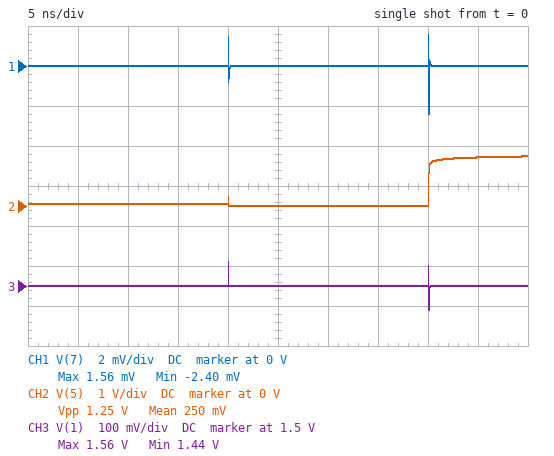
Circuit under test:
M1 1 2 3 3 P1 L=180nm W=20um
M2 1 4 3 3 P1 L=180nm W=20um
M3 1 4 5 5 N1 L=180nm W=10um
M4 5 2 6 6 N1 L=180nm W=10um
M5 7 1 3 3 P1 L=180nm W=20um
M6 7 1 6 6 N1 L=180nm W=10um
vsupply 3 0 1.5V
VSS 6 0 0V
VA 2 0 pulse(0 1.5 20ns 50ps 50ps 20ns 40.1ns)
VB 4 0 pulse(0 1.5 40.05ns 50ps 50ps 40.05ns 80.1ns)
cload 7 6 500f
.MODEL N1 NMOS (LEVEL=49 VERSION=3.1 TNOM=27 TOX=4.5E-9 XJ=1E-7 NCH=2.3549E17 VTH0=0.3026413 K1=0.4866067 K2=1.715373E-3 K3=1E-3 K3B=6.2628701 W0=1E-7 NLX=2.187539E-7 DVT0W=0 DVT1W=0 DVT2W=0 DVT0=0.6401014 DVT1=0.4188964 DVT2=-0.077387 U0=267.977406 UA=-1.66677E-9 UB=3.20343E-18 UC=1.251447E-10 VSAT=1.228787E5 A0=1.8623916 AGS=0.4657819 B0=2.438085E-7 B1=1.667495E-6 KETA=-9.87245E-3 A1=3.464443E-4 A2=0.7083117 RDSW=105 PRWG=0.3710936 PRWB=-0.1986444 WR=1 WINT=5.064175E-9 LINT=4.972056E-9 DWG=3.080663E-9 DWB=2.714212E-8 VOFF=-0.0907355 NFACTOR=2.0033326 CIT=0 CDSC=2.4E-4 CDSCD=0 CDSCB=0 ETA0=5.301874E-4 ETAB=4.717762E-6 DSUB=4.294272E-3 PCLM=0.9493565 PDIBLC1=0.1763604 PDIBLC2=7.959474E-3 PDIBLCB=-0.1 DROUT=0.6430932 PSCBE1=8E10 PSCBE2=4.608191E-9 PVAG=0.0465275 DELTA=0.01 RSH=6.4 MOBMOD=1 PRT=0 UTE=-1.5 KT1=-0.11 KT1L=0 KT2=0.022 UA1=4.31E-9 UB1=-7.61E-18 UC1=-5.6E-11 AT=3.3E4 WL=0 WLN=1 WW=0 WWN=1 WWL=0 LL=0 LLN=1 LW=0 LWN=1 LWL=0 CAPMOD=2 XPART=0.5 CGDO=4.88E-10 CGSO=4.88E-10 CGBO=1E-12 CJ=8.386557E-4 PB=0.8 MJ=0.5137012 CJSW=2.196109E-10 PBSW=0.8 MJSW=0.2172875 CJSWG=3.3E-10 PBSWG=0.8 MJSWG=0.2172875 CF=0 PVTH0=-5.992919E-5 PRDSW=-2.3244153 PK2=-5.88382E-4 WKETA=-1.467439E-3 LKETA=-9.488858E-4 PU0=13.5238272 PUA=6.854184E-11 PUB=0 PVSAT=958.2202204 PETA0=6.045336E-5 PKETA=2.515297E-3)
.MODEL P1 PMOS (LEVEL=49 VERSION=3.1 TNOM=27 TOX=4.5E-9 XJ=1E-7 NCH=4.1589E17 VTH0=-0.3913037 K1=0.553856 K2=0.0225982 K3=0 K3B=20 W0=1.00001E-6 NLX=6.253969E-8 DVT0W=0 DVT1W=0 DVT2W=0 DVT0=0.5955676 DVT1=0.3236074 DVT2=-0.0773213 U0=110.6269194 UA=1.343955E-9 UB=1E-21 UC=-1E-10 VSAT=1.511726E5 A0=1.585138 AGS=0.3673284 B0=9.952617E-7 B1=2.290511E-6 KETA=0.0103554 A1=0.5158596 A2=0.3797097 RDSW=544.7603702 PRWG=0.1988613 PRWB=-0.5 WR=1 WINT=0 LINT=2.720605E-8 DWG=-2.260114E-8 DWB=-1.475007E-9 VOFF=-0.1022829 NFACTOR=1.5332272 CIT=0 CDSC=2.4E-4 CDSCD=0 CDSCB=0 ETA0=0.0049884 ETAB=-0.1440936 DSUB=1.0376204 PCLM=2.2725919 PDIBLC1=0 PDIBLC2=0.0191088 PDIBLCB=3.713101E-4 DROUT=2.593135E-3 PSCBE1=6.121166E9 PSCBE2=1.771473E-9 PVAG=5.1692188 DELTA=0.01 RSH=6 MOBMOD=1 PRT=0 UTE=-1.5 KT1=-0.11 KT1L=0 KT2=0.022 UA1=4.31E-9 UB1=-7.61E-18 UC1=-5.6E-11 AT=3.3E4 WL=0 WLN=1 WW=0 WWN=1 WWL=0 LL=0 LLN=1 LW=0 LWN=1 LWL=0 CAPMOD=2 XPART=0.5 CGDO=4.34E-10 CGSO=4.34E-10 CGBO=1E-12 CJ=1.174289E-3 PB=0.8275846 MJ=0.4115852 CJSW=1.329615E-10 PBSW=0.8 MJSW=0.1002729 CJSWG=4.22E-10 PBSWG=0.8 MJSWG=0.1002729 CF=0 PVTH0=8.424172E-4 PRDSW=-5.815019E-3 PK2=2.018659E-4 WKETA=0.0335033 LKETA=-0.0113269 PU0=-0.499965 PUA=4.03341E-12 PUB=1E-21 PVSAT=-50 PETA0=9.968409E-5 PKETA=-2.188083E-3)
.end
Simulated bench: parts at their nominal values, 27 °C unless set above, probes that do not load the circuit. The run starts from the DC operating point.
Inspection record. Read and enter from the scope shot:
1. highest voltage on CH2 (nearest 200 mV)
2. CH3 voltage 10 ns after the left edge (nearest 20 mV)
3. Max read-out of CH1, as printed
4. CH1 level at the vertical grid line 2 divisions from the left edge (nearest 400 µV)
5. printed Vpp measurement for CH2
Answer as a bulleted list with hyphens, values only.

- 1.2 V
- 1.50 V
- 1.56 mV
- 0 V
- 1.25 V
